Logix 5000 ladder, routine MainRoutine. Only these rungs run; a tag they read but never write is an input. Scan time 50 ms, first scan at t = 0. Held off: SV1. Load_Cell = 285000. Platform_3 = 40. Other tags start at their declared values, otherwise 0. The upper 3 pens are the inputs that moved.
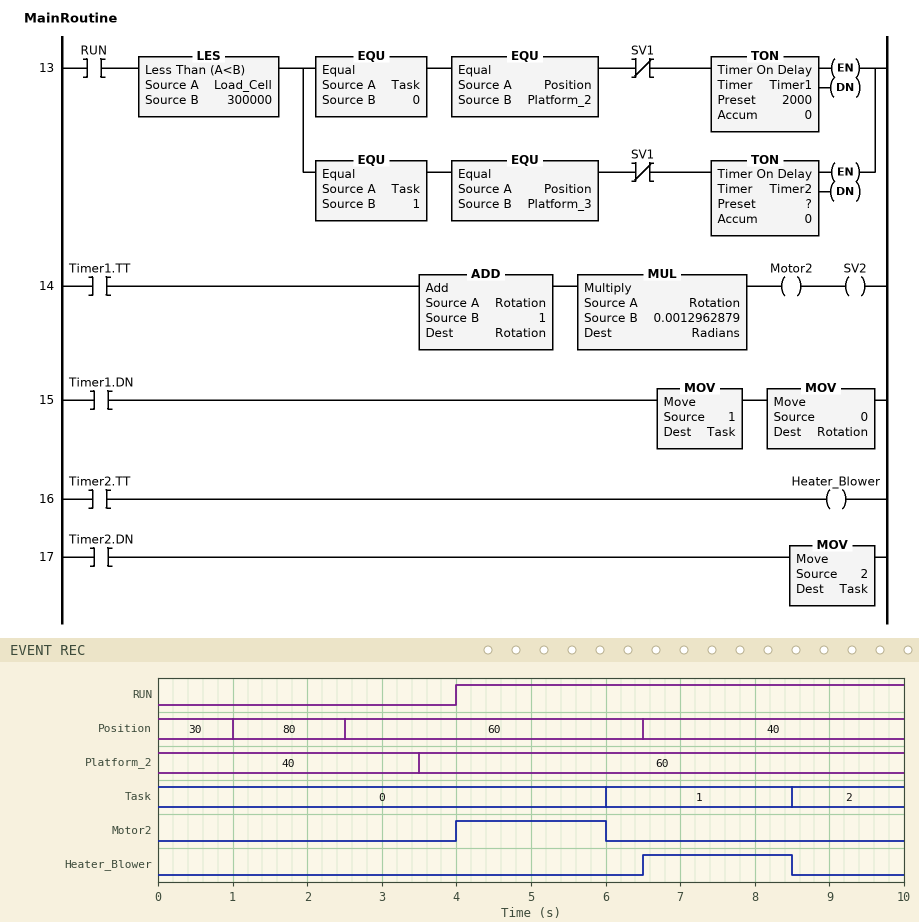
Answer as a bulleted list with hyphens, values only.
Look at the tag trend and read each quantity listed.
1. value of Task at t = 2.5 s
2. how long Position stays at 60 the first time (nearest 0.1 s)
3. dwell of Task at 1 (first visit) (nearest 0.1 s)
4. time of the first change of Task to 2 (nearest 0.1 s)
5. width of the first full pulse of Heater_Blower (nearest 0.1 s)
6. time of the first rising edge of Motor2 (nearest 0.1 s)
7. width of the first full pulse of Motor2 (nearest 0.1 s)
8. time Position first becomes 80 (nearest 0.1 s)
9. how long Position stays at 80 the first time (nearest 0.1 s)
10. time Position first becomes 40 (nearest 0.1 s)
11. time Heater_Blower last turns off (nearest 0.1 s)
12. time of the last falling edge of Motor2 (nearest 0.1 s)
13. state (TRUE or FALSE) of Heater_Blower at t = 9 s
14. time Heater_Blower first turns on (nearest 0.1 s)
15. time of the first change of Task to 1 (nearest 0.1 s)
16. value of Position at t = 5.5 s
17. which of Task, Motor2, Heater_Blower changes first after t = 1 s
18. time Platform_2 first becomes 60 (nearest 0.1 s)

- 0
- 4.0 s
- 2.5 s
- 8.5 s
- 2.0 s
- 4.0 s
- 2.0 s
- 1.0 s
- 1.5 s
- 6.5 s
- 8.5 s
- 6.0 s
- FALSE
- 6.5 s
- 6.0 s
- 60
- Motor2
- 3.5 s
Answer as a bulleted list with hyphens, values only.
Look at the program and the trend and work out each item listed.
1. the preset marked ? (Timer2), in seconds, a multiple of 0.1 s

- 2.0 s
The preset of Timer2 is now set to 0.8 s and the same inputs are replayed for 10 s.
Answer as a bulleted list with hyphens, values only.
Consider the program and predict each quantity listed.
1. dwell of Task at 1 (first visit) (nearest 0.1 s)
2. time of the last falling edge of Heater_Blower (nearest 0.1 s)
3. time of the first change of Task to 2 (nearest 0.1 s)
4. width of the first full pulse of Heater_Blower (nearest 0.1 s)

- 1.3 s
- 7.3 s
- 7.3 s
- 0.8 s
